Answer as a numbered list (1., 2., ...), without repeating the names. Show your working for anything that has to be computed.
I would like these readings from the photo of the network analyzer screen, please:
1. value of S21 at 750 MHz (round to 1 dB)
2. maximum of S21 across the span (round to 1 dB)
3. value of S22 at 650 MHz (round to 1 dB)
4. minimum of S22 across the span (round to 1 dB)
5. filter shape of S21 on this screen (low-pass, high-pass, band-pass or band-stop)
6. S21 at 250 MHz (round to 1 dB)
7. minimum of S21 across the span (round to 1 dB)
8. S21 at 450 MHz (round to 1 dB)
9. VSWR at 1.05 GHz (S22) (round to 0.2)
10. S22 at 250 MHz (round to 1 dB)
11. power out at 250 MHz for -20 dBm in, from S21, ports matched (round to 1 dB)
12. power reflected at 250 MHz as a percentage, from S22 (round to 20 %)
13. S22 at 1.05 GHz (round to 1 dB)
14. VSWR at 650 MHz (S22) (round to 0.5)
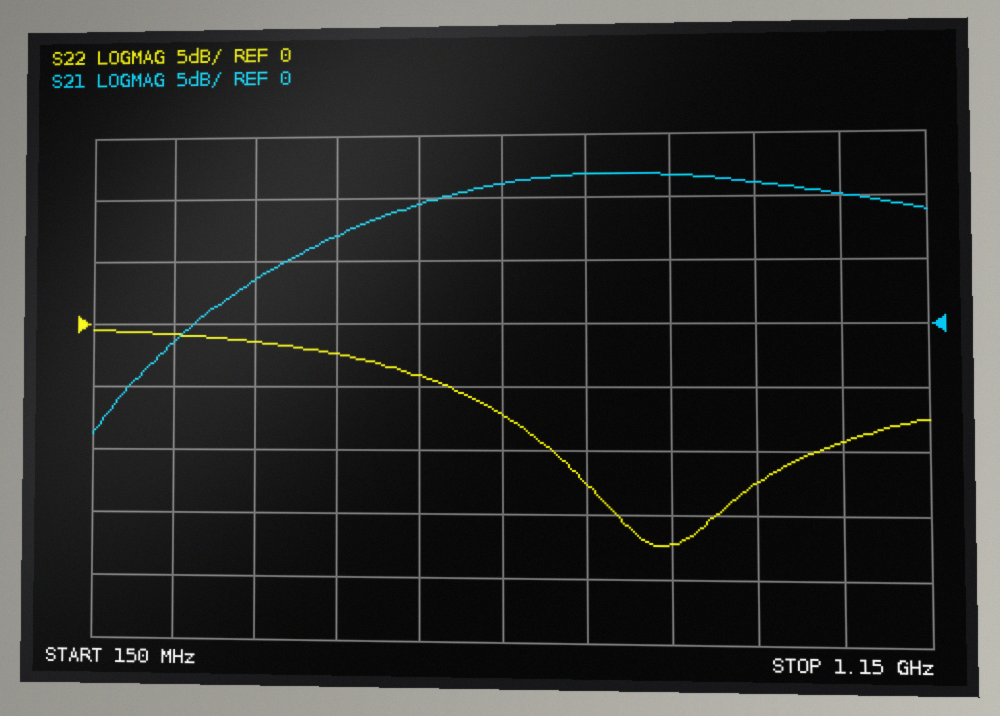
1. 12 dB
2. 12 dB
3. -7 dB
4. -17 dB
5. high-pass
6. -1 dB
7. -9 dB
8. 7 dB
9. |Γ| = 10^(-9/20) = 0.3548; VSWR = (1 + 0.3548)/(1 − 0.3548) ≈ 2.10, so 2.0 to the nearest 0.2
10. -1 dB
11. -20 dBm + (-1 dB) = -21 dBm
12. 10^(-1/10) ≈ 79.4 %, so 80 % to the nearest 20 %
13. -9 dB
14. |Γ| = 10^(-7/20) = 0.4467; VSWR = (1 + 0.4467)/(1 − 0.4467) ≈ 2.61, so 2.5 to the nearest 0.5
